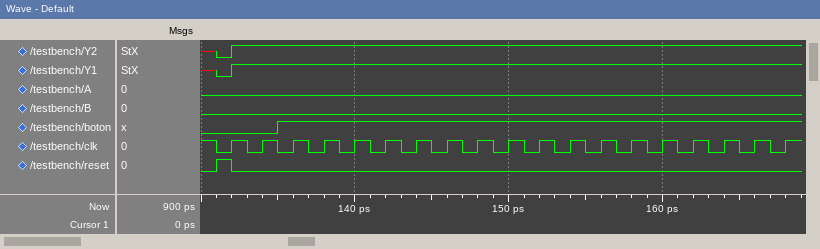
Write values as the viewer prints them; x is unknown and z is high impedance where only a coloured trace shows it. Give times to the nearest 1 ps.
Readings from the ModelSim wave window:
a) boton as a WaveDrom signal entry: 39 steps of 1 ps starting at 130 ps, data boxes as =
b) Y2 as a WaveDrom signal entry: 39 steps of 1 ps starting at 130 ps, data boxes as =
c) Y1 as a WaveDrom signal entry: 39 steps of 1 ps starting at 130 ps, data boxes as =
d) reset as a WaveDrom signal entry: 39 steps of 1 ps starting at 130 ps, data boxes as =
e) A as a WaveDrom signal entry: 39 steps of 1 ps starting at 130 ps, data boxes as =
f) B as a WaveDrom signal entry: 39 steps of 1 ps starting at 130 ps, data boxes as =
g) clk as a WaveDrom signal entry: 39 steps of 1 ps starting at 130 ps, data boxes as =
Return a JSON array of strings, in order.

["{name: 'boton', wave: '0....1.................................'}", "{name: 'Y2', wave: 'x01....................................'}", "{name: 'Y1', wave: 'x01....................................'}", "{name: 'reset', wave: '010....................................'}", "{name: 'A', wave: '0......................................'}", "{name: 'B', wave: '0......................................'}", "{name: 'clk', wave: '101010101010101010101010101010101010101'}"]
